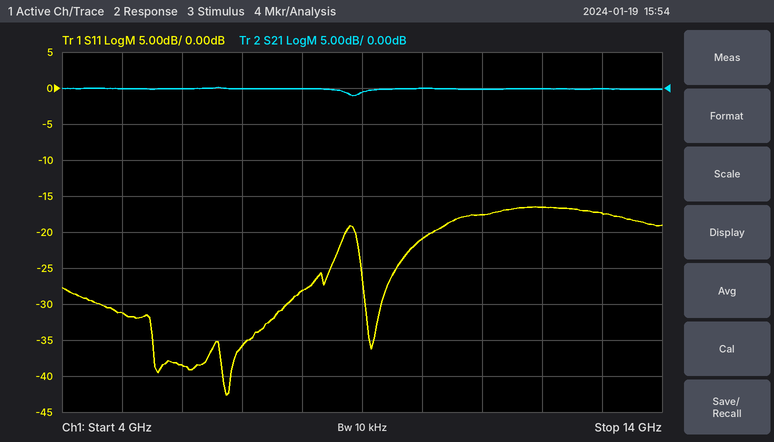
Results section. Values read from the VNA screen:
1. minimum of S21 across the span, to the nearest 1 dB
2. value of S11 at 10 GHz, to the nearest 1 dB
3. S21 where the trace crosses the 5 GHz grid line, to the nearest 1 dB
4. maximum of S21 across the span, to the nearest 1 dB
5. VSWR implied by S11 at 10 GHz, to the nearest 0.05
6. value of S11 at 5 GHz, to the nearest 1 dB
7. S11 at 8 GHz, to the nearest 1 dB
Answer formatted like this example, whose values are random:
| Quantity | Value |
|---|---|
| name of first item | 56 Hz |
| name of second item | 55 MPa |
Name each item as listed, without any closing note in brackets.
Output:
| Quantity | Value |
|---|---|
| minimum of S21 across the span, to the nearest 1 dB | -1 dB |
| value of S11 at 10 GHz, to the nearest 1 dB | -21 dB |
| S21 where the trace crosses the 5 GHz grid line, to the nearest 1 dB | 0 dB |
| maximum of S21 across the span, to the nearest 1 dB | 0 dB |
| VSWR implied by S11 at 10 GHz, to the nearest 0.05 | 1.20 |
| value of S11 at 5 GHz, to the nearest 1 dB | -31 dB |
| S11 at 8 GHz, to the nearest 1 dB | -28 dB |
